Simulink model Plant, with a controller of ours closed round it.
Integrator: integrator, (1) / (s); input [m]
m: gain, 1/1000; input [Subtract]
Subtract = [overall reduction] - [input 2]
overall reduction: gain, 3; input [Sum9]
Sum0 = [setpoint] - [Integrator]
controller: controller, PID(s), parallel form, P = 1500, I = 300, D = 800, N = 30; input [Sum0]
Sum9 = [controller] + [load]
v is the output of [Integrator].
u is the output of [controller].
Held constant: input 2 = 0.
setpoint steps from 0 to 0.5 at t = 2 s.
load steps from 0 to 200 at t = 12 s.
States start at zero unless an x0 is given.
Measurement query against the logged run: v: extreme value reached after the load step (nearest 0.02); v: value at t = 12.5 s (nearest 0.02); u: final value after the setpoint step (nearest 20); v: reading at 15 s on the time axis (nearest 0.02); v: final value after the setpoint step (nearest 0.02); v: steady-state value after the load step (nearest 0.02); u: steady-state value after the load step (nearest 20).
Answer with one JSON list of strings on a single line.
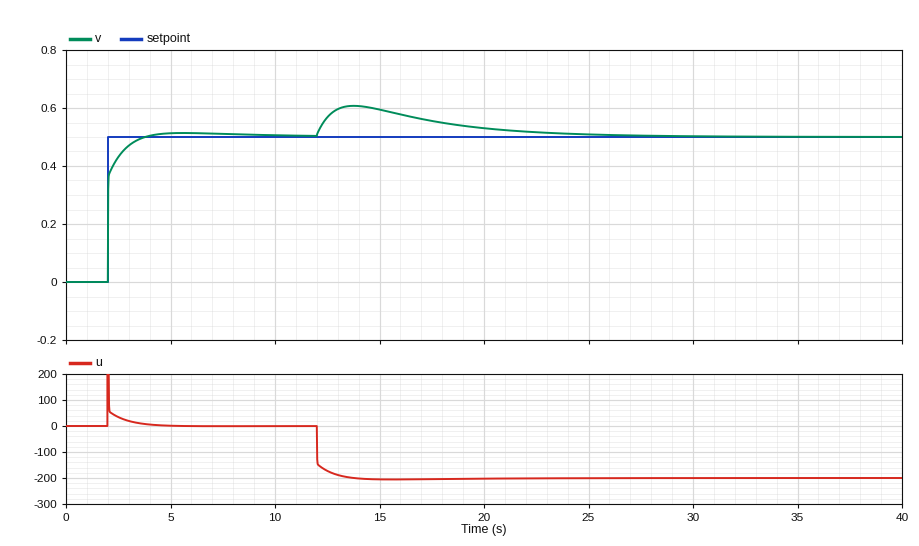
["0.60", "0.56", "0", "0.60", "0.50", "0.50", "-200"]
